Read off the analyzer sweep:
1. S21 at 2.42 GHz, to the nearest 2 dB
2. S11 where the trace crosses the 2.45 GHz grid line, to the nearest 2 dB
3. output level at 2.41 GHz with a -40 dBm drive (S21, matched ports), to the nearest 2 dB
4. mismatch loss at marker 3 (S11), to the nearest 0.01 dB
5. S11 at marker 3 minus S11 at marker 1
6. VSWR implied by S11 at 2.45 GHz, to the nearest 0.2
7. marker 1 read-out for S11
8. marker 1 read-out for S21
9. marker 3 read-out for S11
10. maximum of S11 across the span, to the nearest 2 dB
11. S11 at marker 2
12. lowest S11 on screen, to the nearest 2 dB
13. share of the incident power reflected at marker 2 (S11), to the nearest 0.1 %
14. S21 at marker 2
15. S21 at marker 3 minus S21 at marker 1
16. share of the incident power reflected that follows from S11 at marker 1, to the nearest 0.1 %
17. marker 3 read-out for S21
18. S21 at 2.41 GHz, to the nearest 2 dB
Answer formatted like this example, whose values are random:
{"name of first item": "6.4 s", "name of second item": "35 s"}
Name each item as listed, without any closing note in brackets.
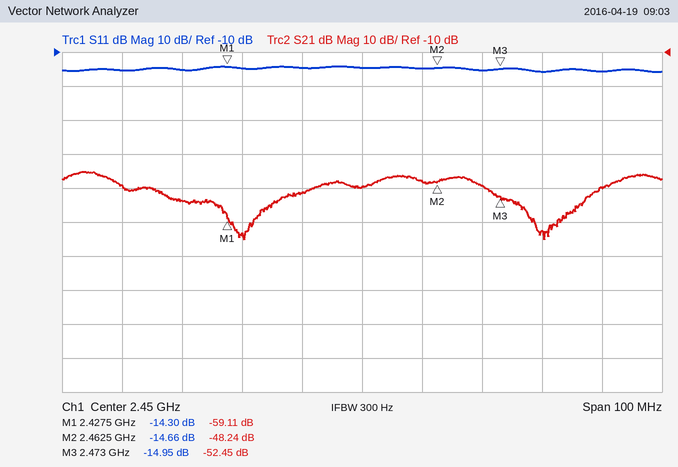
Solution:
{"S21 at 2.42 GHz, to the nearest 2 dB": "-54 dB", "S11 where the trace crosses the 2.45 GHz grid line, to the nearest 2 dB": "-14 dB", "output level at 2.41 GHz with a -40 dBm drive (S21, matched ports), to the nearest 2 dB": "-90 dBm", "mismatch loss at marker 3 (S11), to the nearest 0.01 dB": "0.14 dB", "S11 at marker 3 minus S11 at marker 1": "-0.65 dB", "VSWR implied by S11 at 2.45 GHz, to the nearest 0.2": "1.4", "marker 1 read-out for S11": "-14.30 dB", "marker 1 read-out for S21": "-59.11 dB", "marker 3 read-out for S11": "-14.95 dB", "maximum of S11 across the span, to the nearest 2 dB": "-14 dB", "S11 at marker 2": "-14.66 dB", "lowest S11 on screen, to the nearest 2 dB": "-16 dB", "share of the incident power reflected at marker 2 (S11), to the nearest 0.1 %": "3.4 %", "S21 at marker 2": "-48.24 dB", "S21 at marker 3 minus S21 at marker 1": "6.66 dB", "share of the incident power reflected that follows from S11 at marker 1, to the nearest 0.1 %": "3.7 %", "marker 3 read-out for S21": "-52.45 dB", "S21 at 2.41 GHz, to the nearest 2 dB": "-50 dB"}
